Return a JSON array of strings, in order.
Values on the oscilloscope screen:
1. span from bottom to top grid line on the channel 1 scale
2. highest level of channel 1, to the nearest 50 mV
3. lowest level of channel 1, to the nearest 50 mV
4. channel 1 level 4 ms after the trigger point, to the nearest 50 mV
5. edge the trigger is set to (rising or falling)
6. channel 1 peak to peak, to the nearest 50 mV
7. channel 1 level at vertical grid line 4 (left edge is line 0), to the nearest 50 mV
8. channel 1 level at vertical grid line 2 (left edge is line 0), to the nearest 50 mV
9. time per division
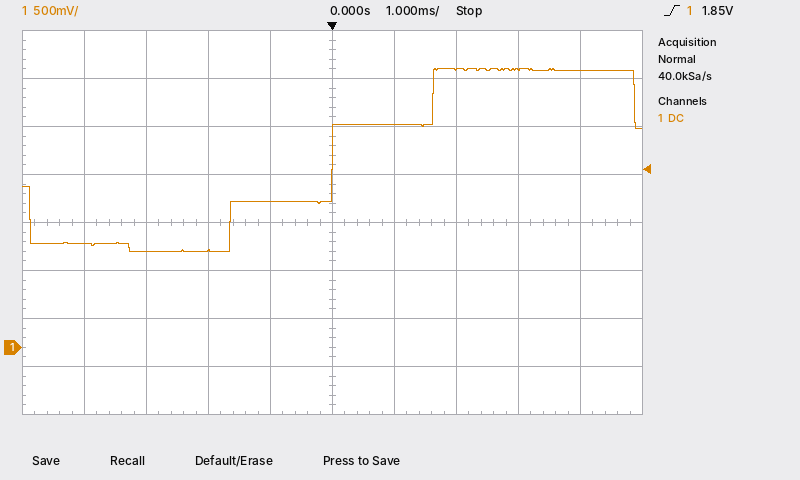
["4 V", "2.90 V", "1.00 V", "2.90 V", "rising", "1.90 V", "1.50 V", "1.00 V", "1 ms"]
